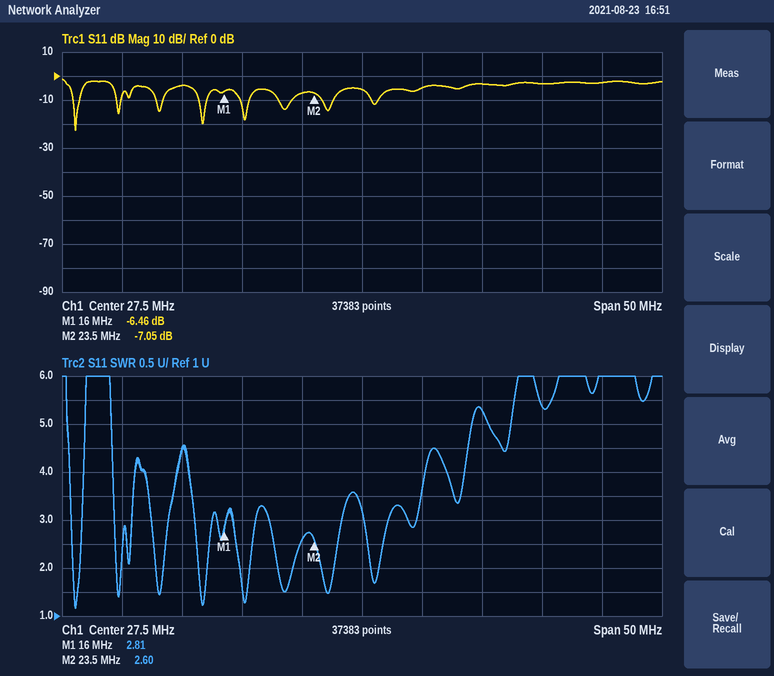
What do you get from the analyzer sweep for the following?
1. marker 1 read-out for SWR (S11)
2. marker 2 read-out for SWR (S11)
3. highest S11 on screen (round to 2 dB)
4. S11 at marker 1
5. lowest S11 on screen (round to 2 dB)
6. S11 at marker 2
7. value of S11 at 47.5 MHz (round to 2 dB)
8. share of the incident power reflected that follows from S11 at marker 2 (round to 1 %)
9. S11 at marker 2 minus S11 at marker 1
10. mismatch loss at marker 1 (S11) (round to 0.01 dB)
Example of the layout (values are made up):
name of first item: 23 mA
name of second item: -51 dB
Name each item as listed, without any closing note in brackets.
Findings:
marker 1 read-out for SWR: 2.81
marker 2 read-out for SWR: 2.60
highest S11 on screen: -2 dB
S11 at marker 1: -6.46 dB
lowest S11 on screen: -22 dB
S11 at marker 2: -7.05 dB
value of S11 at 47.5 MHz: -2 dB
share of the incident power reflected that follows from S11 at marker 2: 20 %
S11 at marker 2 minus S11 at marker 1: -0.59 dB
mismatch loss at marker 1 (S11): 1.11 dB
